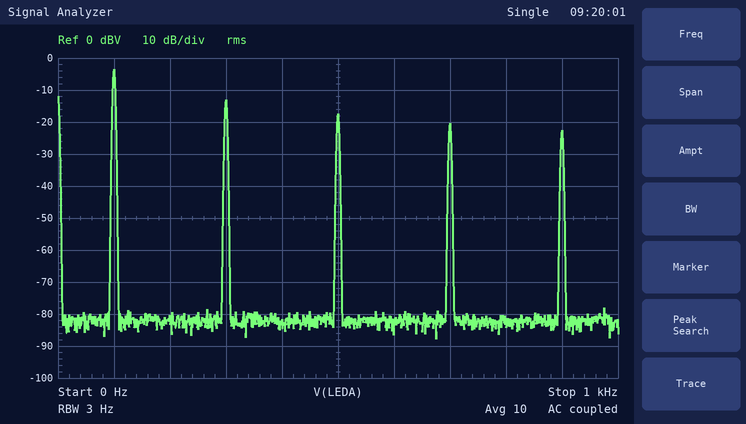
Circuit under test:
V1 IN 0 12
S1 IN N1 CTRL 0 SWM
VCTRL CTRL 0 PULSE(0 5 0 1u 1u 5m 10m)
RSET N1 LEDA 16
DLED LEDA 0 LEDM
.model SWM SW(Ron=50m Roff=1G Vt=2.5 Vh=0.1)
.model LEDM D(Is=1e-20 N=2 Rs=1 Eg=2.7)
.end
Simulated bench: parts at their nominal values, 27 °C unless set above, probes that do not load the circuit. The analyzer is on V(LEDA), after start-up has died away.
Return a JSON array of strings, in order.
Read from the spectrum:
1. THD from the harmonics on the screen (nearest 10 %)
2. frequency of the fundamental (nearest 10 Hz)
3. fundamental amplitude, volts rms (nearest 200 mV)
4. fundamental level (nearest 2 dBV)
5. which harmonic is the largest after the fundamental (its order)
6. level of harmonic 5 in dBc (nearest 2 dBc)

["40 %", "100 Hz", "600 mV", "-4 dBV", "3", "-14 dBc"]
